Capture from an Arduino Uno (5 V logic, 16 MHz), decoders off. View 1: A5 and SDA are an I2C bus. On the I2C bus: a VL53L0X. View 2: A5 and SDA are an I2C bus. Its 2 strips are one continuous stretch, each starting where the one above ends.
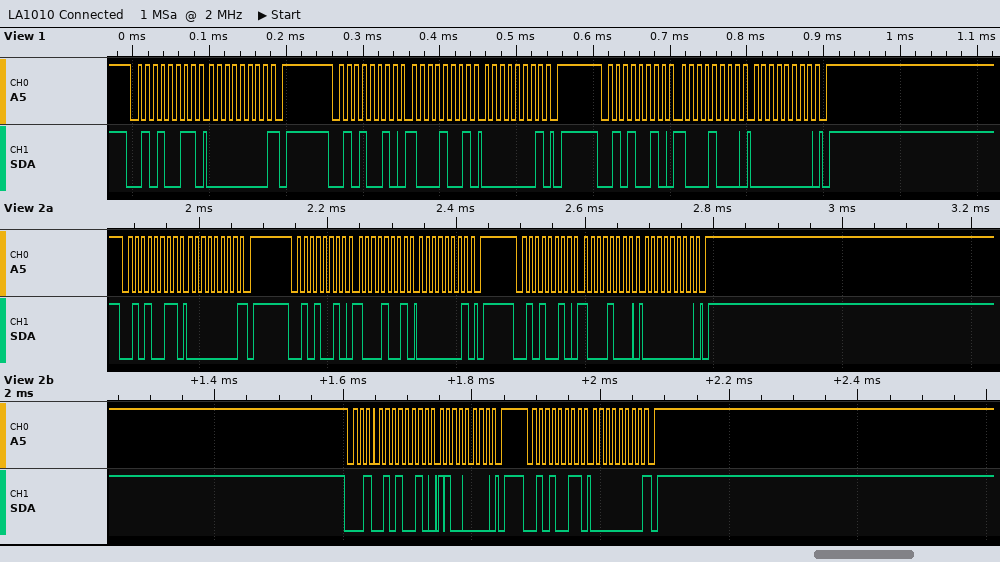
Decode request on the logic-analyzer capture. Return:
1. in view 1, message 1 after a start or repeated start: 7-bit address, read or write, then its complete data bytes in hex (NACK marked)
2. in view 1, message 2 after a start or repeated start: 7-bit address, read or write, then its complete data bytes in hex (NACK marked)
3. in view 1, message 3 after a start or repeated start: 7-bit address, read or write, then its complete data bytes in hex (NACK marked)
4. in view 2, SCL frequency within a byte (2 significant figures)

0x29 read: 00 NACK
0x29 write: 89 01
0x29 write: 88 00
100 kHz
